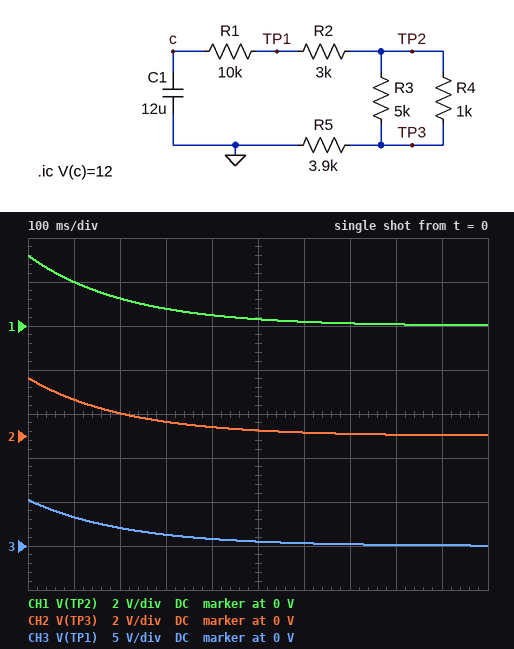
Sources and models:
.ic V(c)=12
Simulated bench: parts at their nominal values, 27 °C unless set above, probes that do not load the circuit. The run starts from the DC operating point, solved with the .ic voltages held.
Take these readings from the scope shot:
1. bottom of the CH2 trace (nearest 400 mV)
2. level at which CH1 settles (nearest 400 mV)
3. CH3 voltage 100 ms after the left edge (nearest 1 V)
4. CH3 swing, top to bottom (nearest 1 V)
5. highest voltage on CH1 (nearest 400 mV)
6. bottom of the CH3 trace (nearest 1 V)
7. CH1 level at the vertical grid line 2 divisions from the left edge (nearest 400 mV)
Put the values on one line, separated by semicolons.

0 V; 0 V; 3 V; 5 V; 3.2 V; 0 V; 1.2 V
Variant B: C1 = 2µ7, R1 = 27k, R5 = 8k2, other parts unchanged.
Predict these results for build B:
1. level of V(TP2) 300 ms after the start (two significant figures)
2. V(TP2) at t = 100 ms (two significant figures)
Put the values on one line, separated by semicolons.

160 mV; 1.1 V
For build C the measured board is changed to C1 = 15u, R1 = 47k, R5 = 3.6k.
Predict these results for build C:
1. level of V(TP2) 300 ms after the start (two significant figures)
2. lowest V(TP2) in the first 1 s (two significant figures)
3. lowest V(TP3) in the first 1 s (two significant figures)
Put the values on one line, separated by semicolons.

680 mV; 290 mV; 230 mV
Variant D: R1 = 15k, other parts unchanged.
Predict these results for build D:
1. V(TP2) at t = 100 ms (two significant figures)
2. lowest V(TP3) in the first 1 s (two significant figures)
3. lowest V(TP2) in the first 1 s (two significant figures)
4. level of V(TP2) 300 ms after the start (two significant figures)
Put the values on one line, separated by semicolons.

1.7 V; 53 mV; 64 mV; 830 mV
